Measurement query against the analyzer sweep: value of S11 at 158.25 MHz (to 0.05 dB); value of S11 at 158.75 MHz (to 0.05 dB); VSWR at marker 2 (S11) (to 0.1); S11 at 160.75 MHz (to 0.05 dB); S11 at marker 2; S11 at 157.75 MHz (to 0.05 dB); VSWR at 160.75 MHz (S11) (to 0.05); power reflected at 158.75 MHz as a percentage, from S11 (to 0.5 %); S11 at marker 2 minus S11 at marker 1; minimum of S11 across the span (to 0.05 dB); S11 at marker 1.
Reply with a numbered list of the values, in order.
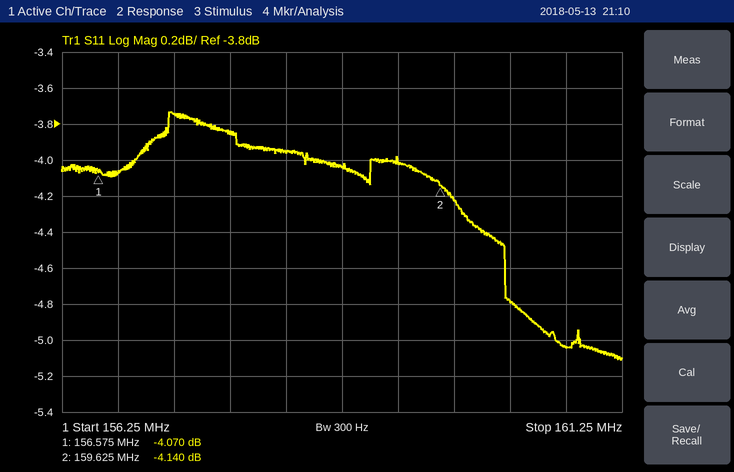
1. -3.95 dB
2. -4.05 dB
3. 4.3
4. -5.05 dB
5. -4.140 dB
6. -3.85 dB
7. 3.55
8. 39.5 %
9. -0.070 dB
10. -5.10 dB
11. -4.070 dB
